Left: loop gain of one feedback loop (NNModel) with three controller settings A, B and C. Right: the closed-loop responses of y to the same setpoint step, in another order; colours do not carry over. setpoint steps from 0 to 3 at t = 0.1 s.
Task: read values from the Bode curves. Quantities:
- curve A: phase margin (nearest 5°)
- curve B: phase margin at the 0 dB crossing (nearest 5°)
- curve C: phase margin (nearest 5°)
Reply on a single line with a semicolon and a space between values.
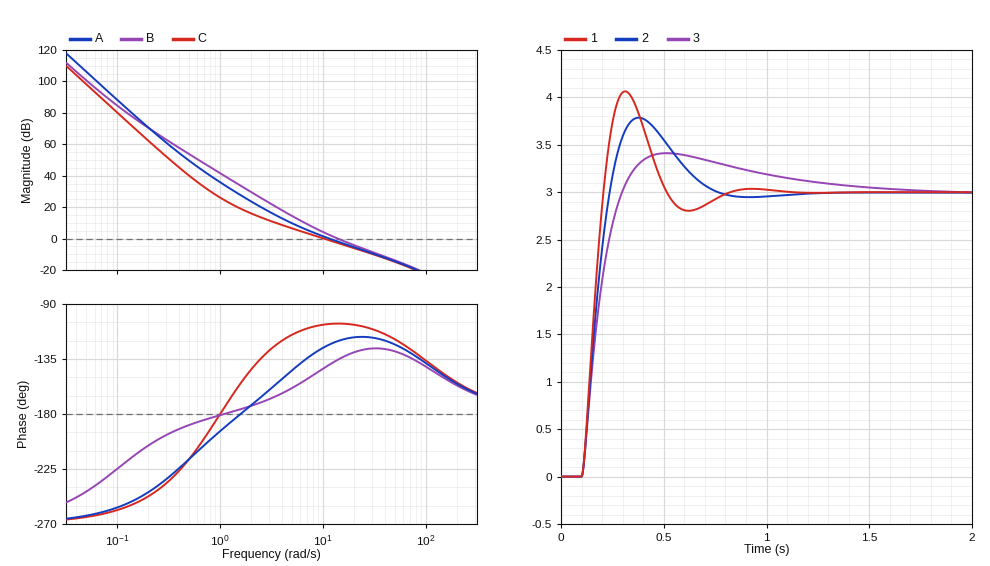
55°; 45°; 75°
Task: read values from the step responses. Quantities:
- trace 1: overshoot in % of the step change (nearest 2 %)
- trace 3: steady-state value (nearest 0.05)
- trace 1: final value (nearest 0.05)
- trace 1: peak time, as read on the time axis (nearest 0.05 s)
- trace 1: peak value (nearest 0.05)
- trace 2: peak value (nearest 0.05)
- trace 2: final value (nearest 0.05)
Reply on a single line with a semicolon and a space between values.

36 %; 3.00; 3.00; 0.30 s; 4.05; 3.80; 3.00
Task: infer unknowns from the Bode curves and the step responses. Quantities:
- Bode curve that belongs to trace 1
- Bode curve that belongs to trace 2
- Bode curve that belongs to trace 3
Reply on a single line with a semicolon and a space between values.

B; A; C
